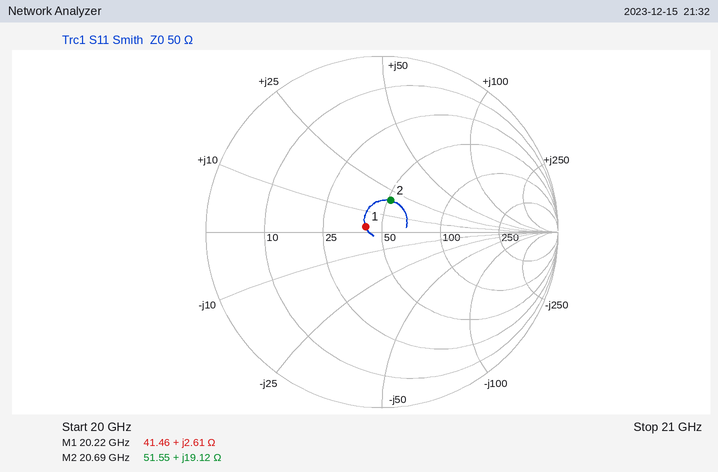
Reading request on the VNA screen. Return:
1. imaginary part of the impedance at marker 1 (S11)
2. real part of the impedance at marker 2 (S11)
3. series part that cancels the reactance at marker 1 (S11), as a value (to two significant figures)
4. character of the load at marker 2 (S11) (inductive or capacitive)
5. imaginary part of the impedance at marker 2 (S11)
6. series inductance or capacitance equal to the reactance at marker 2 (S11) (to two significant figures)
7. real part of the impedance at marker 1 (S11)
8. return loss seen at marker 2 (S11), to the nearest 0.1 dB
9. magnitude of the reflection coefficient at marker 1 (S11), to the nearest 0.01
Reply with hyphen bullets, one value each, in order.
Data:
- +2.61 Ω
- 51.55 Ω
- 3.0 pF
- inductive
- +19.12 Ω
- 150 pH
- 41.46 Ω
- 14.6 dB
- 0.10
